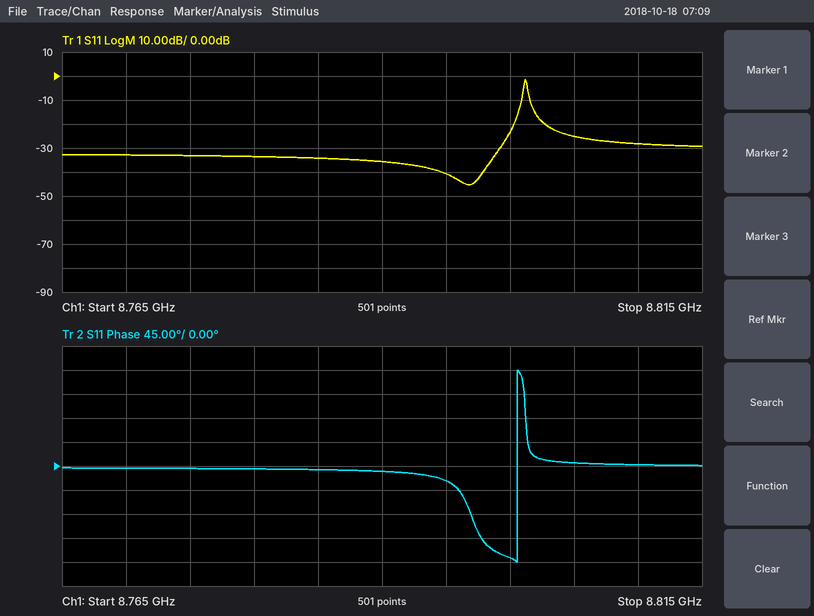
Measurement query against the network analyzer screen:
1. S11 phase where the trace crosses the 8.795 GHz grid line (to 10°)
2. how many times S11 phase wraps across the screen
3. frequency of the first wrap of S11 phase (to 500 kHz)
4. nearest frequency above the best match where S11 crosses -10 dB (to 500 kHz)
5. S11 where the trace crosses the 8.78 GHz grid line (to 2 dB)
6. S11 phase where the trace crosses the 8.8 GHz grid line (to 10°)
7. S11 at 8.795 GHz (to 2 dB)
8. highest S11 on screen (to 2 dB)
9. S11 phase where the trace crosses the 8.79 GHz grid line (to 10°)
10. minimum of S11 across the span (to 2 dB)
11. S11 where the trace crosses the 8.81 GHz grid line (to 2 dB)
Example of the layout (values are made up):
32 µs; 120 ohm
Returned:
-30°; 1; 8.8005 GHz; 8.8010 GHz; -34 dB; -170°; -40 dB; -2 dB; -10°; -46 dB; -28 dB
